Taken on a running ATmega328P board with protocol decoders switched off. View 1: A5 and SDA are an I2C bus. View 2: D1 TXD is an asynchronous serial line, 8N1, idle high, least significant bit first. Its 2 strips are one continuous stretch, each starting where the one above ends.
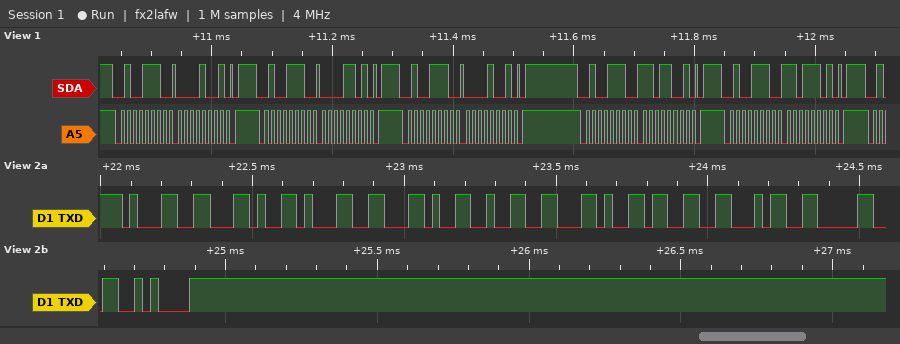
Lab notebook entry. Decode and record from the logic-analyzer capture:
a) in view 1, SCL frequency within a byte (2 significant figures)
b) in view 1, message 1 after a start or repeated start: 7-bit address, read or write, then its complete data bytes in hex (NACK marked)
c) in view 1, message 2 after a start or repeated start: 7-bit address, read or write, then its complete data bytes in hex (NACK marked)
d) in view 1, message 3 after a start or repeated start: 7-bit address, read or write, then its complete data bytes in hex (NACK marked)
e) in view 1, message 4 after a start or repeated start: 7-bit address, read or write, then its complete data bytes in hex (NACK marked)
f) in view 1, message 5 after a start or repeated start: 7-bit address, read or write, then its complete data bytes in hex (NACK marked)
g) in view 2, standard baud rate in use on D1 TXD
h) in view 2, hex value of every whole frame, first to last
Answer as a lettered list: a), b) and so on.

a) 100 kHz
b) 0x27 write: 09
c) 0x27 write: 0D
d) 0x27 write: 09
e) 0x27 write: D9
f) 0x27 write: DD
g) 38400 baud
h) 0x31 0x2C 0x31 0x2C 0x32 0x2C 0x33 0x34 0x30 0x0A
